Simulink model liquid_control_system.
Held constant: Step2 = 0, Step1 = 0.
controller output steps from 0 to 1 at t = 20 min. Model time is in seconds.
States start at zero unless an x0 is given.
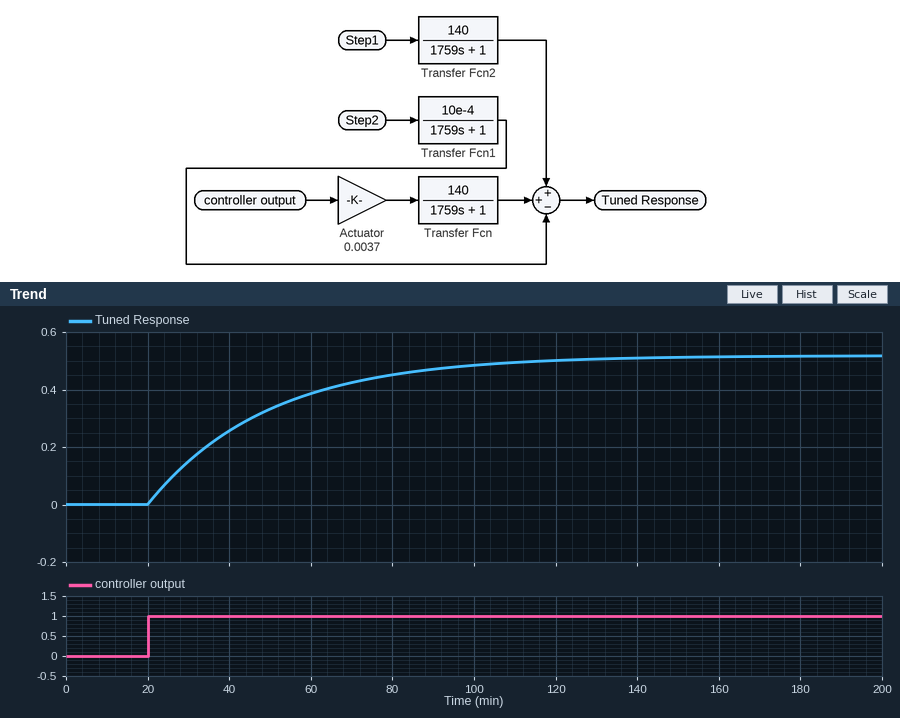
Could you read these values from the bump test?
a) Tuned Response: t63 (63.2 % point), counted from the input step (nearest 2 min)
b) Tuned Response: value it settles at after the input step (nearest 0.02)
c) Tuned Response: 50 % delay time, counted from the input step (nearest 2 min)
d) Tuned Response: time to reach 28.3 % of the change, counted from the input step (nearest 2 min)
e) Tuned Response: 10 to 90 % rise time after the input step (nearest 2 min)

30 min
0.52
20 min
10 min
64 min
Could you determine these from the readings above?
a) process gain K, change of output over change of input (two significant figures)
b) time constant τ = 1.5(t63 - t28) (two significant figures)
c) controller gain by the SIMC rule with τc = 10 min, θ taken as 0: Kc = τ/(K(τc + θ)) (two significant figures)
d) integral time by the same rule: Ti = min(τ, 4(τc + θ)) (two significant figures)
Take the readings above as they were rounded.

0.52
30 min
5.8
30 min
